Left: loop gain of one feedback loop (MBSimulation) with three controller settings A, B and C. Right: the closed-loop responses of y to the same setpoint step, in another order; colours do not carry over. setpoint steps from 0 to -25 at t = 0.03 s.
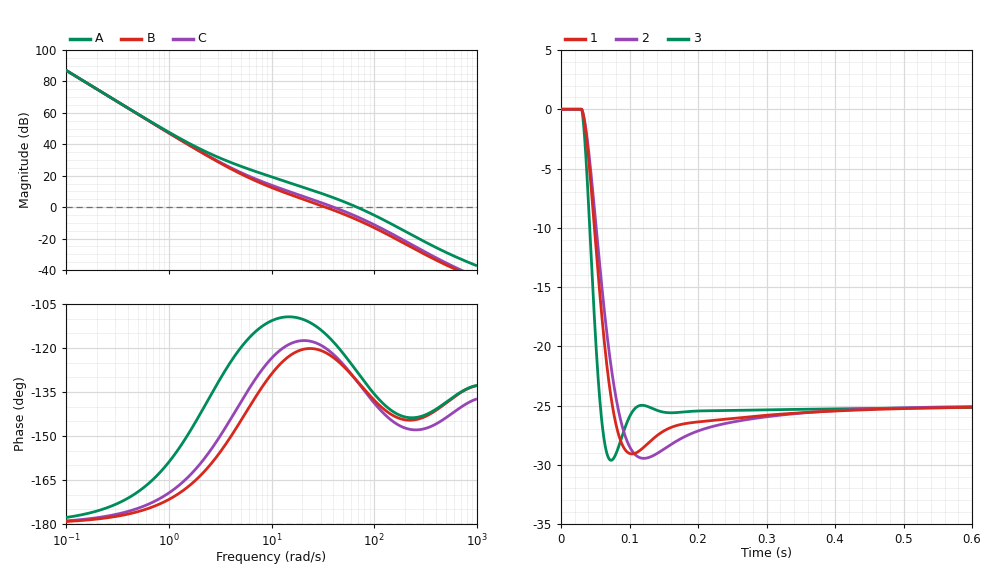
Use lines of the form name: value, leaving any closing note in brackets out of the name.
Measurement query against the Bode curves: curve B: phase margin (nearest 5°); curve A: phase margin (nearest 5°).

curve B: phase margin: 60°
curve A: phase margin: 50°
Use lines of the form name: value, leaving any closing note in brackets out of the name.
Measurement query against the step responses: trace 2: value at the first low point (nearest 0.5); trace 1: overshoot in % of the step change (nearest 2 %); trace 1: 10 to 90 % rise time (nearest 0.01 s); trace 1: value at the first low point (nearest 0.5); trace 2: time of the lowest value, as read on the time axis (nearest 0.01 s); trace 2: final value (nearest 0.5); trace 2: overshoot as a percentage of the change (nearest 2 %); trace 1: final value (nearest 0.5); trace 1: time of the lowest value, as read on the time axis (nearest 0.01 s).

trace 2: value at the first low point: -29.5
trace 1: overshoot in % of the step change: 16 %
trace 1: 10 to 90 % rise time: 0.03 s
trace 1: value at the first low point: -29.0
trace 2: time of the lowest value, as read on the time axis: 0.12 s
trace 2: final value: -25.0
trace 2: overshoot as a percentage of the change: 18 %
trace 1: final value: -25.0
trace 1: time of the lowest value, as read on the time axis: 0.10 s
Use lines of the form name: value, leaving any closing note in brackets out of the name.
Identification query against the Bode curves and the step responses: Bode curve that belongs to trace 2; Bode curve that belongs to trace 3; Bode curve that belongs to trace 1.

Bode curve that belongs to trace 2: B
Bode curve that belongs to trace 3: A
Bode curve that belongs to trace 1: C
